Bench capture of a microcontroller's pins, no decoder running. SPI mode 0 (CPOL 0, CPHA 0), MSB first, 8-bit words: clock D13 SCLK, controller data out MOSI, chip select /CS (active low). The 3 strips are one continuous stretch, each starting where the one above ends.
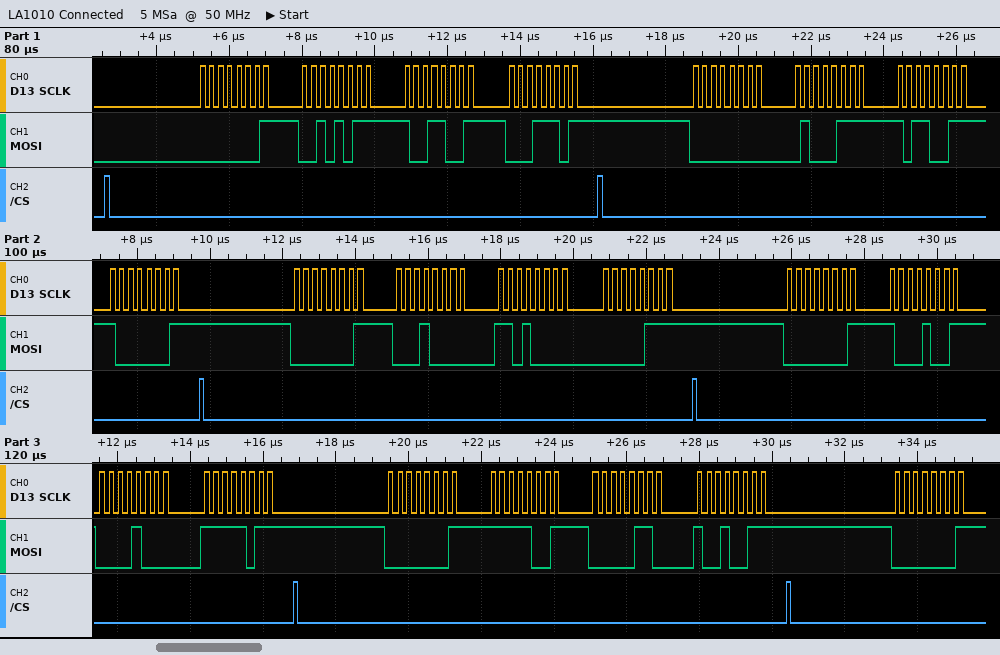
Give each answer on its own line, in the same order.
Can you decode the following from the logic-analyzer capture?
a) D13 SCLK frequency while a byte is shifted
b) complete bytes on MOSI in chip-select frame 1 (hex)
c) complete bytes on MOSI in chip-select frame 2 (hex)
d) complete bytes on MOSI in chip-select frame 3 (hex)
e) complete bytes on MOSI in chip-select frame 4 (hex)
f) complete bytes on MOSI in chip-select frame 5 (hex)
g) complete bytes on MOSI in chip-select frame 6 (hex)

4 MHz
0x01 0x2B 0x99 0x1D
0x00 0x47 0xB3 0x81
0x01 0x10 0xD0 0x07
0x01 0x89 0x08 0xFB
0x01 0xF9 0x06 0x93
0x01
